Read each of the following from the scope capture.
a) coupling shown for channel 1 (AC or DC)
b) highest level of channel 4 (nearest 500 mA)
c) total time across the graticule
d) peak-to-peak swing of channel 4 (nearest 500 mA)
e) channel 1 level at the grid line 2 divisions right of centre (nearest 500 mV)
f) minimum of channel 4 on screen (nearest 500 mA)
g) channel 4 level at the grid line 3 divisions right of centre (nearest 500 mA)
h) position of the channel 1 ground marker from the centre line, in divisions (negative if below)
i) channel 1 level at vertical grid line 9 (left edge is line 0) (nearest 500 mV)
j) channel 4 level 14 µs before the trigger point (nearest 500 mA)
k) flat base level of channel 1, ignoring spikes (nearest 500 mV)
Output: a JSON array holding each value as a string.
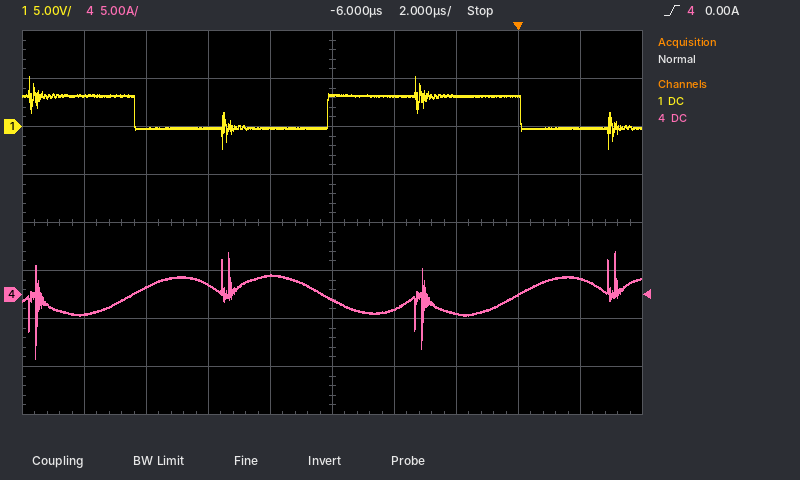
["DC", "4.5 A", "20 µs", "11.0 A", "3.0 V", "-6.5 A", "0.0 A", "+2.0 div", "0.0 V", "-2.0 A", "0.0 V"]
